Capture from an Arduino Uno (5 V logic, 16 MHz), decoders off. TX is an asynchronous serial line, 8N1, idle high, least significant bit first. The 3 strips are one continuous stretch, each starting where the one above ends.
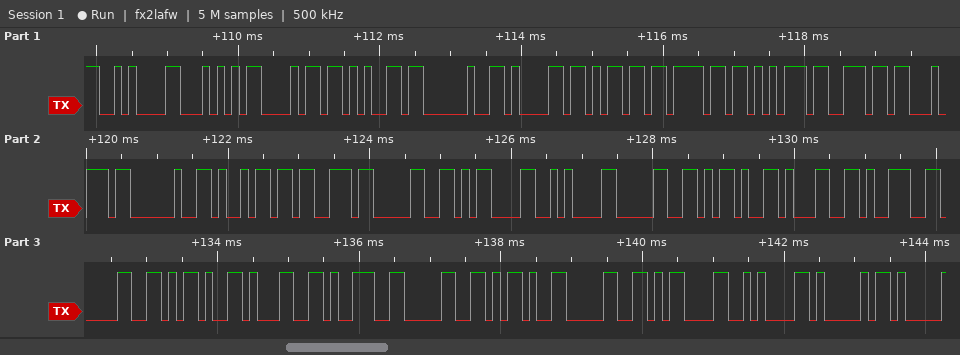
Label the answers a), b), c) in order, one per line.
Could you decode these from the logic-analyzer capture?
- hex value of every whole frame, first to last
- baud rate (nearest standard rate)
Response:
a) 0A 54 68 65 20 61 6D 6F 75 6E 74 20 69 73 30 0D 0A 30 2D 31 39 30 2D 31 39 30 2D 30 0D 0A 41
b) 9600 baud
